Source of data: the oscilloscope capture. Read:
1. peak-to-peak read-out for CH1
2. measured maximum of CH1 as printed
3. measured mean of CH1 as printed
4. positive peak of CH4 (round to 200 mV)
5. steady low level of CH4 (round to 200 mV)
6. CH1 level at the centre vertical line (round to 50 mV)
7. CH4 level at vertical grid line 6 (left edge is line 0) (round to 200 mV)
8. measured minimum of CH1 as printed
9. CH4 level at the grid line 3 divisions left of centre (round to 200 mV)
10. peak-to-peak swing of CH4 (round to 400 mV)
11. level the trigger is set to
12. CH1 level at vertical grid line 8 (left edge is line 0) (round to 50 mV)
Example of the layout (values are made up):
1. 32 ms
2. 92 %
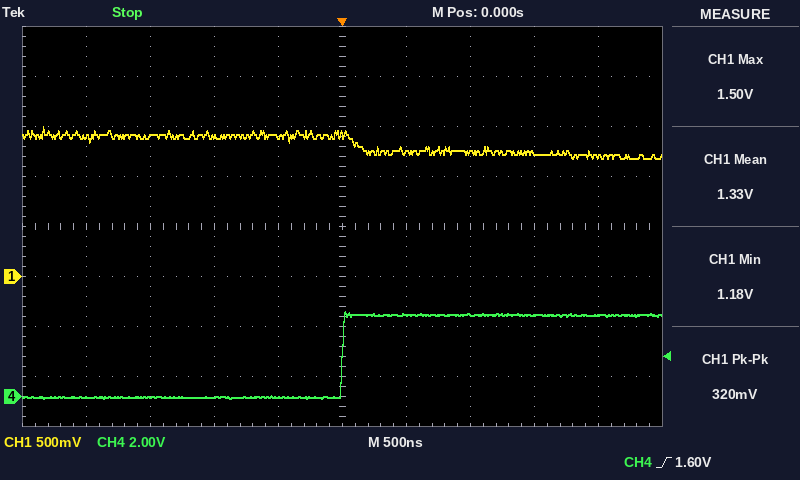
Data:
1. 320 mV
2. 1.50 V
3. 1.33 V
4. 3.4 V
5. 0.0 V
6. 1.40 V
7. 3.2 V
8. 1.18 V
9. 0.0 V
10. 3.6 V
11. 1.60 V
12. 1.25 V
